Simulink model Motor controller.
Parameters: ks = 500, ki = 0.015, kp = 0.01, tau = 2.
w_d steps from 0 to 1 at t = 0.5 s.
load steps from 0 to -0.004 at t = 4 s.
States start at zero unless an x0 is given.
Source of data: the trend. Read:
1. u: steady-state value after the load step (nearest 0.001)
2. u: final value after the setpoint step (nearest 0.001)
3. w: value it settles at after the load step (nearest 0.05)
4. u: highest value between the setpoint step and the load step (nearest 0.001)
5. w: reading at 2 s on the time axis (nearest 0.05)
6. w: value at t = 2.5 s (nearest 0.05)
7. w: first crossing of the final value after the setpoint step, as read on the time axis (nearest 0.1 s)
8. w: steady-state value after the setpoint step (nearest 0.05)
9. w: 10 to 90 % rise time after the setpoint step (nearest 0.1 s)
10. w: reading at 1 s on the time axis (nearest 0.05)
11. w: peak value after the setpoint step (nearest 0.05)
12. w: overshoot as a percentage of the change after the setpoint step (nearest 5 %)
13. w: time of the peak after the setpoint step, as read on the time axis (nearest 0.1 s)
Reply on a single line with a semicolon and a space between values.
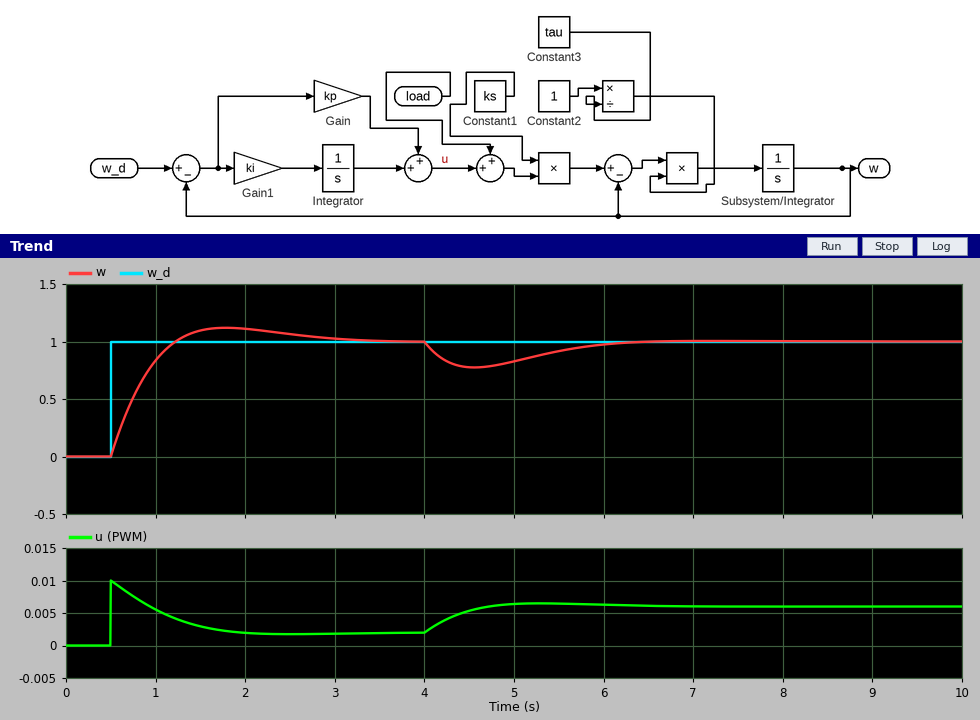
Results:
0.006; 0.002; 1.00; 0.010; 1.10; 1.05; 1.2 s; 1.00; 0.5 s; 0.85; 1.10; 10 %; 1.8 s
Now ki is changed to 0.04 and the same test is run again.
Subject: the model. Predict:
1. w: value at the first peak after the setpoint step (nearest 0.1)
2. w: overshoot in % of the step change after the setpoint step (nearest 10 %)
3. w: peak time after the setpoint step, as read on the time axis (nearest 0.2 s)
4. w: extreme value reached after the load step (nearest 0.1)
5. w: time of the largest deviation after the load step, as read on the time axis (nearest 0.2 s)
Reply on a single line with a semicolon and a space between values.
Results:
1.3; 30 %; 1.4 s; 0.8; 4.4 s
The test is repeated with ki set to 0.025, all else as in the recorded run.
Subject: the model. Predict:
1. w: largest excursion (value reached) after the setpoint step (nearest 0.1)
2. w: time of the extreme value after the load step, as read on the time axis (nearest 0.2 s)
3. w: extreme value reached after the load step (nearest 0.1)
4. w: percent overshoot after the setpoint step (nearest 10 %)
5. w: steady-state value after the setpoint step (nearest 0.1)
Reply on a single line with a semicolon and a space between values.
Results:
1.2; 4.4 s; 0.8; 20 %; 1.0
